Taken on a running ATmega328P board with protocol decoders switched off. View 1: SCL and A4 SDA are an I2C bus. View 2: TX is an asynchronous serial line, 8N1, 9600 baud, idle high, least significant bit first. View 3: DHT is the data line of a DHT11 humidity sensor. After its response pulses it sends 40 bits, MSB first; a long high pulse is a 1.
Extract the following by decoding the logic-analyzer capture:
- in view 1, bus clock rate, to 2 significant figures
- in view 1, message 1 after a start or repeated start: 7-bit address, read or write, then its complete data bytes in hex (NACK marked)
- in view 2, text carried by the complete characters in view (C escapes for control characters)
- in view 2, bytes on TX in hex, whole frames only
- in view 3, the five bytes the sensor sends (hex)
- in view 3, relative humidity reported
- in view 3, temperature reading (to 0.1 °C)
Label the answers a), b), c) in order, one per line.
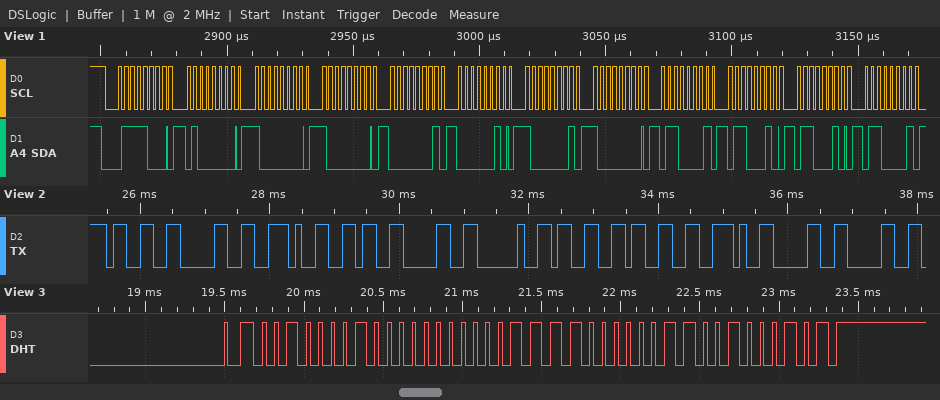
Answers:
a) 400 kHz
b) 0x3C write: 40 80 80 01 02 81 80 61 62 62 61
c) "30.60 33.00"
d) 0x33 0x30 0x2E 0x36 0x30 0x20 0x33 0x33 0x2E 0x30 0x30
e) 21 00 1E 06 45
f) 33 %
g) 30.6 °C
